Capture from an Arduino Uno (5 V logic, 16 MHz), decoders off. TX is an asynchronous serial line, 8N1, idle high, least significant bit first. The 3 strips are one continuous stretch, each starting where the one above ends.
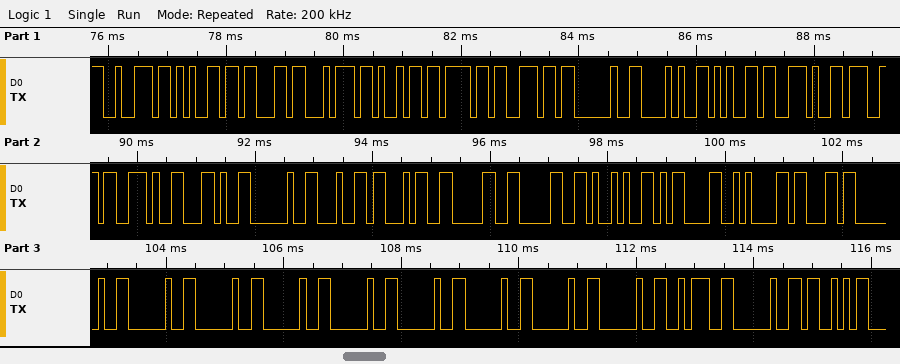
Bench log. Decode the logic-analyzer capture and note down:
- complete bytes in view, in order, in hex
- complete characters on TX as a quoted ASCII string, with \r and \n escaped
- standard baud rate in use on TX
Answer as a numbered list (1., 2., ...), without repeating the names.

1. 72 65 63 74 69 6F 6E 20 28 65 2E 67 2E 2C 20 64 34 30 30 29 0D 0A 63 20 20 20 20 20 20 20 20 20 3A 20 53
2. "rection (e.g., d400)\r\nc         : S"
3. 9600 baud
